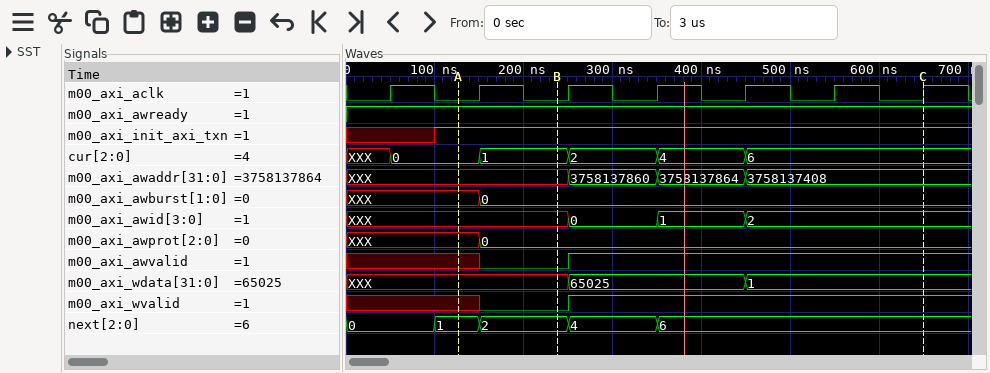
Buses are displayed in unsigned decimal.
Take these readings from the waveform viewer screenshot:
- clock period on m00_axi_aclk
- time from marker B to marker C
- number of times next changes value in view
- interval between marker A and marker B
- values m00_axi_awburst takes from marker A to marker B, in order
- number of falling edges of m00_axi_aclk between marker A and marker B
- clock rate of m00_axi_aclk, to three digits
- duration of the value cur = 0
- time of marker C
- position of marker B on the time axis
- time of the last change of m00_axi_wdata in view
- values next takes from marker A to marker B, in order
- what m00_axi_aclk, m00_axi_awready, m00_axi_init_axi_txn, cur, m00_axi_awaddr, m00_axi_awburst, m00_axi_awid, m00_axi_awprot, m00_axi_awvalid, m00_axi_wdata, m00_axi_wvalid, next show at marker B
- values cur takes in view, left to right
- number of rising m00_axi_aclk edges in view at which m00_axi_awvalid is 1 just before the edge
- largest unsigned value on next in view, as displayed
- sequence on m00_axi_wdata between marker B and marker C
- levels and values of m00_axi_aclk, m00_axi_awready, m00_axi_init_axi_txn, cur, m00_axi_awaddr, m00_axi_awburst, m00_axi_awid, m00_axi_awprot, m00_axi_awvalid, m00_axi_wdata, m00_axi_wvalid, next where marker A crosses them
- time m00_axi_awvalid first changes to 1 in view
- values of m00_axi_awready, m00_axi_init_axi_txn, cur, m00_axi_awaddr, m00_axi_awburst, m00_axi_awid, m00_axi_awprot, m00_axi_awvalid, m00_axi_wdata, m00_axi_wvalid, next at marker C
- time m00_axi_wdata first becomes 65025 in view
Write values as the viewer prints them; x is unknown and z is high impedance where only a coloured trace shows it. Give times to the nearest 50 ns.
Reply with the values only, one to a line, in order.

100 ns
400 ns
4
100 ns
XXX, 0
1
10.0 MHz
100 ns
650 ns
250 ns
450 ns
1, 2
m00_axi_aclk=0, m00_axi_awready=1, m00_axi_init_axi_txn=1, cur=1, m00_axi_awaddr=XXX, m00_axi_awburst=0, m00_axi_awid=XXX, m00_axi_awprot=0, m00_axi_awvalid=0, m00_axi_wdata=XXX, m00_axi_wvalid=0, next=2
XXX, 0, 1, 2, 4, 6
4
6
XXX, 65025, 1
m00_axi_aclk=0, m00_axi_awready=1, m00_axi_init_axi_txn=1, cur=0, m00_axi_awaddr=XXX, m00_axi_awburst=XXX, m00_axi_awid=XXX, m00_axi_awprot=XXX, m00_axi_awvalid=x, m00_axi_wdata=XXX, m00_axi_wvalid=x, next=1
250 ns
m00_axi_awready=1, m00_axi_init_axi_txn=1, cur=6, m00_axi_awaddr=3758137408, m00_axi_awburst=0, m00_axi_awid=2, m00_axi_awprot=0, m00_axi_awvalid=1, m00_axi_wdata=1, m00_axi_wvalid=1, next=6
250 ns
